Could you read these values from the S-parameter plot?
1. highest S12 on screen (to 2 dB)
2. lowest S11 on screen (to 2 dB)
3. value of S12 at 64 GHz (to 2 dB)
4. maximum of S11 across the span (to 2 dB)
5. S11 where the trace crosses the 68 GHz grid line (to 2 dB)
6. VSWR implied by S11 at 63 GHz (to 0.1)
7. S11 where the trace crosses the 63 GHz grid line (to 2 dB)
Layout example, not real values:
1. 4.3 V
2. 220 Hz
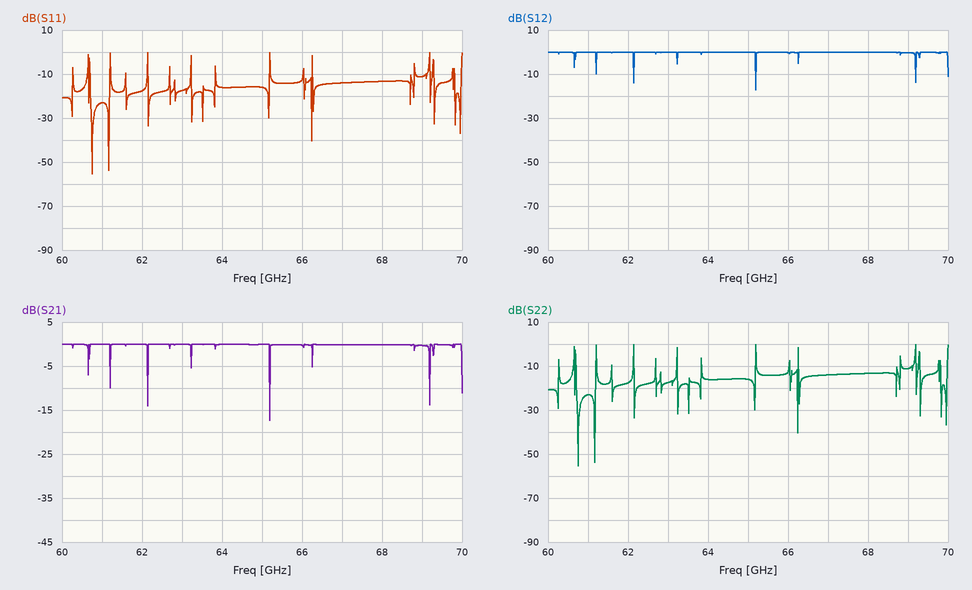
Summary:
1. 0 dB
2. -56 dB
3. 0 dB
4. 0 dB
5. -14 dB
6. 1.3
7. -18 dB
